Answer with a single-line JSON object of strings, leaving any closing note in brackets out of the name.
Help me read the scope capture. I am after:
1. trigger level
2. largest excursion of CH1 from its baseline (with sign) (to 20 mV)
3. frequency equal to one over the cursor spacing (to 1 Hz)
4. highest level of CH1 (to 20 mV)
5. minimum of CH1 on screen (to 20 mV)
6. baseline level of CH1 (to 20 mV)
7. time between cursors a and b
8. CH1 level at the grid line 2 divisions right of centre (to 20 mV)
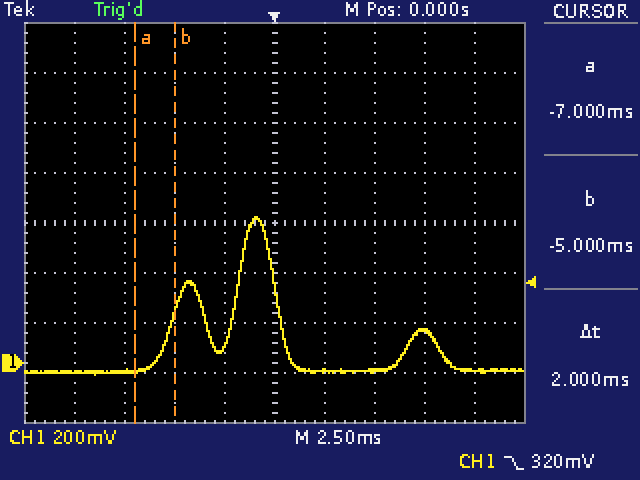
{"trigger level": "320 mV", "largest excursion of CH1 from its baseline (with sign)": "+620 mV", "frequency equal to one over the cursor spacing": "500 Hz", "highest level of CH1": "580 mV", "minimum of CH1 on screen": "-40 mV", "baseline level of CH1": "-40 mV", "time between cursors a and b": "2 ms", "CH1 level at the grid line 2 divisions right of centre": "-40 mV"}
